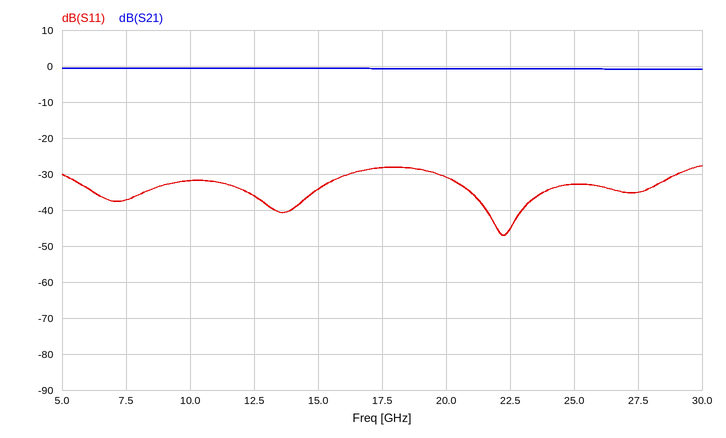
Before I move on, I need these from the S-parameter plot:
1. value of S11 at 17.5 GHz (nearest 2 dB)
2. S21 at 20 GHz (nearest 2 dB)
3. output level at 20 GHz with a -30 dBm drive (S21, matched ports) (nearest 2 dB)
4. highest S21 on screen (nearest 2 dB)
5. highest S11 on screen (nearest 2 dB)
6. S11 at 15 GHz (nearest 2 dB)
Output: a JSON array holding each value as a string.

["-28 dB", "0 dB", "-30 dBm", "0 dB", "-28 dB", "-34 dB"]
